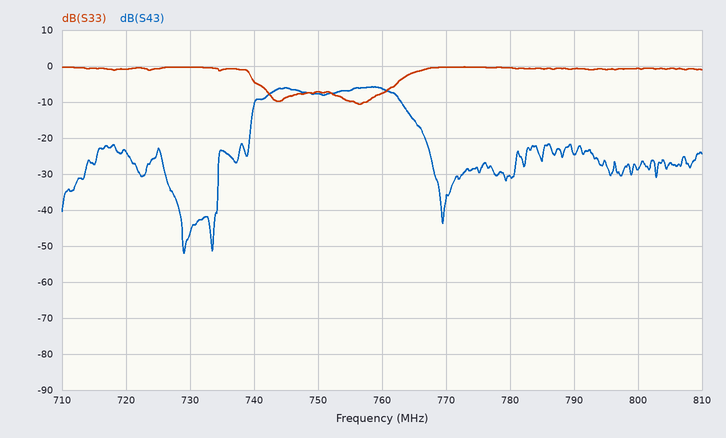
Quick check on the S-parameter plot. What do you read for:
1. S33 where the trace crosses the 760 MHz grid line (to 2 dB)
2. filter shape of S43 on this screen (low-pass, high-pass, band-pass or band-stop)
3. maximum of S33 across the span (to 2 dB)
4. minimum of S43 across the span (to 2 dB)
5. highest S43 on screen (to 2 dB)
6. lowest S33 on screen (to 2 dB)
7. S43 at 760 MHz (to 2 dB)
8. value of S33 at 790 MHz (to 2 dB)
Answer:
-8 dB
band-pass
0 dB
-52 dB
-6 dB
-10 dB
-6 dB
0 dB
